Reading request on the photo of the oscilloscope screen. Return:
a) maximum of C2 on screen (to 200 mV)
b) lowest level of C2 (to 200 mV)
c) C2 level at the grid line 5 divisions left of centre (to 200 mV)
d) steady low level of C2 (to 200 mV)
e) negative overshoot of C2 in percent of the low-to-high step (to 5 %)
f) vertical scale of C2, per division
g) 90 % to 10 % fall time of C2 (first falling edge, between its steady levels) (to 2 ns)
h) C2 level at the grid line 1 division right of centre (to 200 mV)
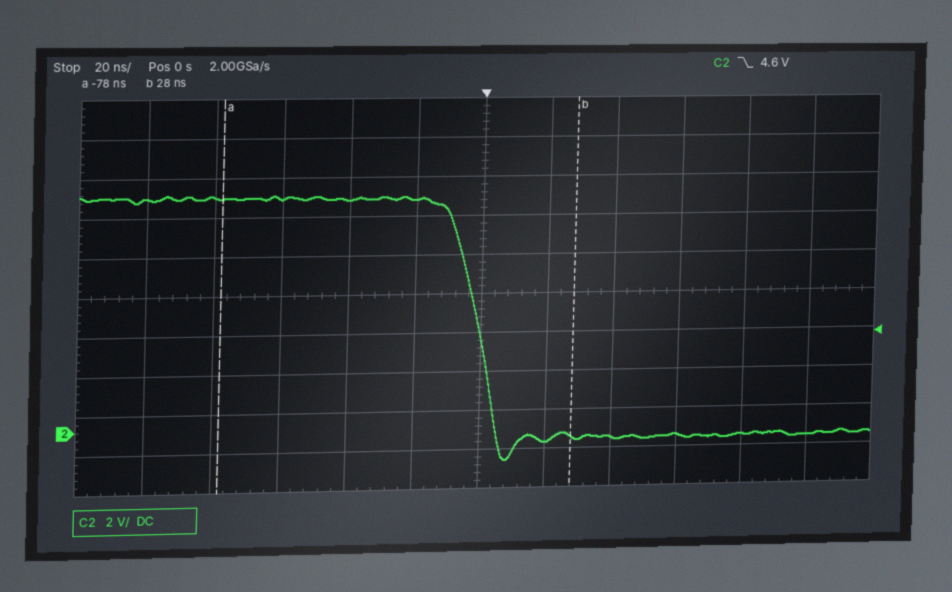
12.0 V
-1.8 V
11.8 V
-600 mV
10 %
2 V
14 ns
-800 mV
